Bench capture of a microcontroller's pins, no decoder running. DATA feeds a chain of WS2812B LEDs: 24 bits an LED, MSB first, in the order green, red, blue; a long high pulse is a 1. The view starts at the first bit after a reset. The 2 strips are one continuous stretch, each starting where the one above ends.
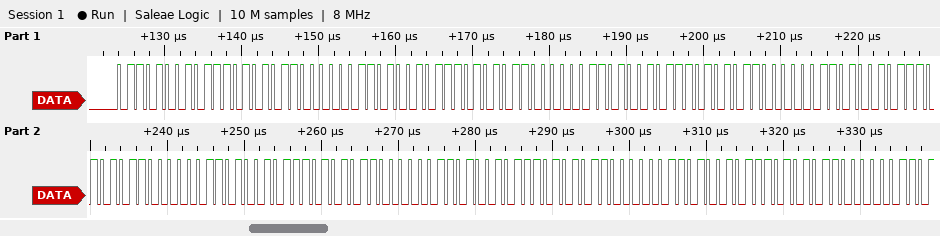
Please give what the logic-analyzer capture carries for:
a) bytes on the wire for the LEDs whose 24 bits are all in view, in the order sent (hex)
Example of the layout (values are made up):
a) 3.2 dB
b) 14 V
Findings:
a) 69 75 60 69 75 60 69 75 60 69 75 60 69 75 60 69 75 60 69 75 60
